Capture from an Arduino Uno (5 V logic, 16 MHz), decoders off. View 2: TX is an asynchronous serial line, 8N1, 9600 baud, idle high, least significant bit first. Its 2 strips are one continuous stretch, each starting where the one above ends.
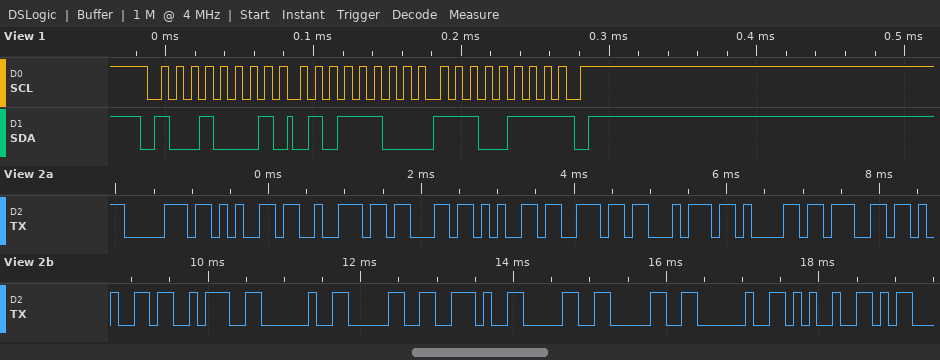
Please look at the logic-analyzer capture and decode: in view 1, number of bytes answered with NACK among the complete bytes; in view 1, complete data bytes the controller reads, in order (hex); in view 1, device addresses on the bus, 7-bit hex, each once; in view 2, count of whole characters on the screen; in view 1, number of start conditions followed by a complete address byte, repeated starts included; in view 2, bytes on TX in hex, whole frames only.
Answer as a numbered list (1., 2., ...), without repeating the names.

1. 1
2. 5C E7
3. 0x48
4. 18
5. 1
6. 0x70 0x65 0x72 0x63 0x65 0x6E 0x74 0x61 0x67 0x65 0x3A 0x20 0x30 0x2E 0x30 0x30 0x20 0x25
